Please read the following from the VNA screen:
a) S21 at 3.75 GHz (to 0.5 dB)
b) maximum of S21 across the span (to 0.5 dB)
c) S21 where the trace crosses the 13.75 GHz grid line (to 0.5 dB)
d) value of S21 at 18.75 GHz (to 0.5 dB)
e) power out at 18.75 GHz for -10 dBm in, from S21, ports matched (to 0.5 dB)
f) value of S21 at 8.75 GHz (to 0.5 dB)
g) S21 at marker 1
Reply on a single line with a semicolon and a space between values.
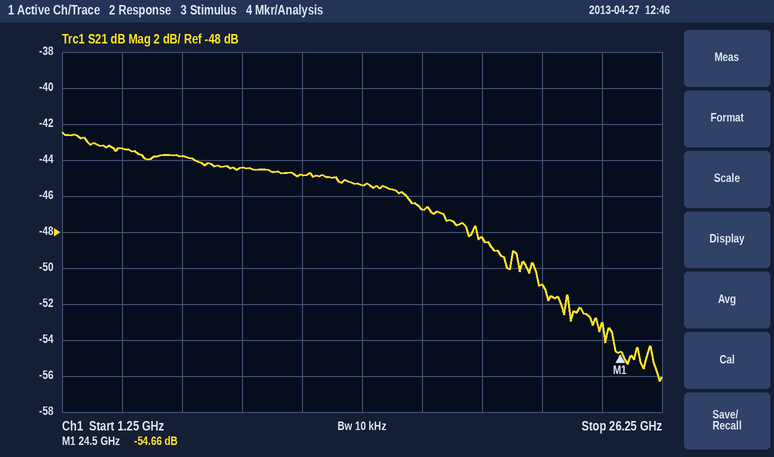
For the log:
-43.5 dB; -42.5 dB; -45.5 dB; -48.5 dB; -58.5 dBm; -44.5 dB; -54.66 dB
